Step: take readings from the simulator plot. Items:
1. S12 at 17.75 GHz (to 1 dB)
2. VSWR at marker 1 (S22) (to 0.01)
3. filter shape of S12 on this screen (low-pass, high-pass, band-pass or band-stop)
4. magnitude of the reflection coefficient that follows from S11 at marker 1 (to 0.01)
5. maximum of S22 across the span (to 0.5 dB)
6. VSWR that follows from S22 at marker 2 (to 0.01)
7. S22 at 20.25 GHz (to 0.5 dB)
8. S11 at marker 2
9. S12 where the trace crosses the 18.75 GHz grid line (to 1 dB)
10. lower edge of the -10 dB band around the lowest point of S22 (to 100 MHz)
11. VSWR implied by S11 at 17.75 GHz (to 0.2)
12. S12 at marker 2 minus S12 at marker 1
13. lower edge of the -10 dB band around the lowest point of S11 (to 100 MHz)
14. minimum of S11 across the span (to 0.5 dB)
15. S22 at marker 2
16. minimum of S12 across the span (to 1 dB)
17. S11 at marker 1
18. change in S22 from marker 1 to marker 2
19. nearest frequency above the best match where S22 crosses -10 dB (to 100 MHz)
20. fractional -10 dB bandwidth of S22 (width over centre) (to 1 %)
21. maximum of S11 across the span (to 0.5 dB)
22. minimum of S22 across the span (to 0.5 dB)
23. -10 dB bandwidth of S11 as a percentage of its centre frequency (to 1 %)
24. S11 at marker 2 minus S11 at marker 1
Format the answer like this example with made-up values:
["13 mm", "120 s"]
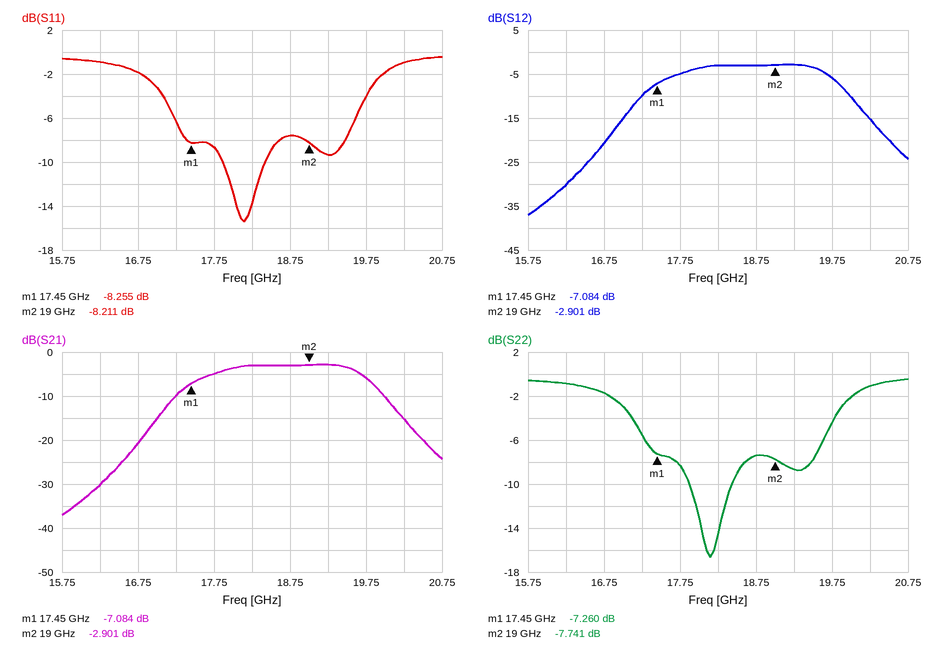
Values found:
["-5 dB", "2.53", "band-pass", "0.39", "-0.5 dB", "2.39", "-1.0 dB", "-8.211 dB", "-3 dB", "17.9 GHz", "2.2", "4.183 dB", "17.9 GHz", "-15.5 dB", "-7.741 dB", "-37 dB", "-8.255 dB", "-0.481 dB", "18.4 GHz", "3 %", "-0.5 dB", "-16.5 dB", "3 %", "0.044 dB"]
